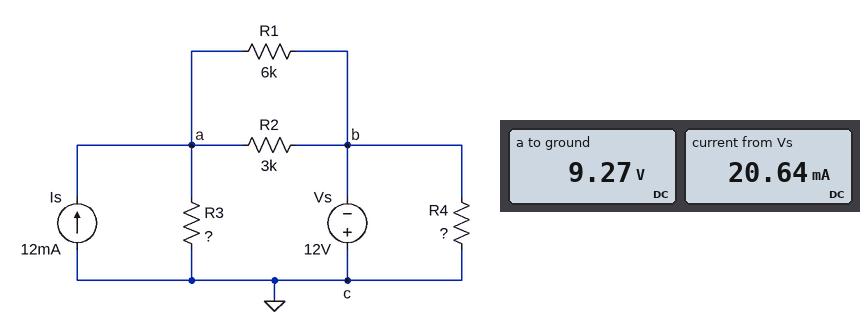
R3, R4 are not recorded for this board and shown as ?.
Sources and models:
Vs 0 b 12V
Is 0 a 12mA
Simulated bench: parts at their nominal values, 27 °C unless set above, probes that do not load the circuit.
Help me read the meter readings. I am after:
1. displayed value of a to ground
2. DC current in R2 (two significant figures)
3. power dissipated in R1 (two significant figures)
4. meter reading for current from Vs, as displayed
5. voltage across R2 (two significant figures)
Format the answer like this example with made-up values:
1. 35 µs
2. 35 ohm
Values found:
1. 9.27 V
2. 7.1 mA
3. 75 mW
4. 20.64 mA
5. 21 V
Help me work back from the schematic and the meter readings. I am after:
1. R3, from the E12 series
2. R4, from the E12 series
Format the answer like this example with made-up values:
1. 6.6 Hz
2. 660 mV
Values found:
1. 6.8 kΩ
2. 1.2 kΩ
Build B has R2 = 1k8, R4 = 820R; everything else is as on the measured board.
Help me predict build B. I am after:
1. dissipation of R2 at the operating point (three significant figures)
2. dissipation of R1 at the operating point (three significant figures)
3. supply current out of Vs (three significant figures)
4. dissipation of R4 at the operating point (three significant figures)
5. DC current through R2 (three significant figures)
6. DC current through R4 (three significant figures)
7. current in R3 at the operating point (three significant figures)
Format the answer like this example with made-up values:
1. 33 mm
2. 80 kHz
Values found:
1. 139 mW
2. 41.8 mW
3. 26.1 mA
4. 176 mW
5. 8.80 mA
6. 14.6 mA
7. 564 µA
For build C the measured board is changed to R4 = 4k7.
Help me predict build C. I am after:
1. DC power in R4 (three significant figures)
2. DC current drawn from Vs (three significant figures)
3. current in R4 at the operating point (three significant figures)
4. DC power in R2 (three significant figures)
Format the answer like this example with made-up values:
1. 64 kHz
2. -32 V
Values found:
1. 30.6 mW
2. 13.2 mA
3. 2.55 mA
4. 151 mW
